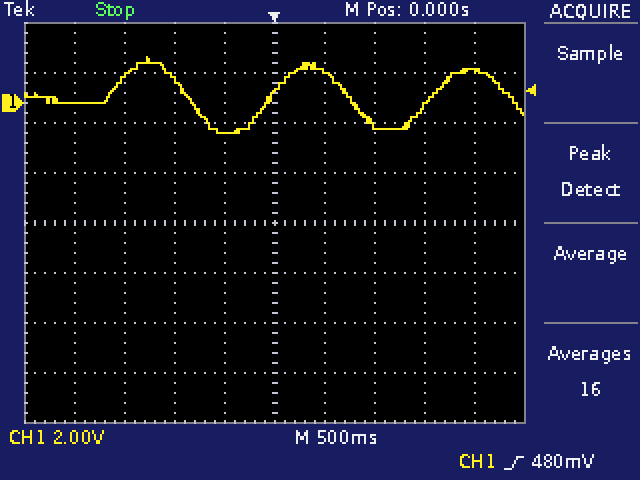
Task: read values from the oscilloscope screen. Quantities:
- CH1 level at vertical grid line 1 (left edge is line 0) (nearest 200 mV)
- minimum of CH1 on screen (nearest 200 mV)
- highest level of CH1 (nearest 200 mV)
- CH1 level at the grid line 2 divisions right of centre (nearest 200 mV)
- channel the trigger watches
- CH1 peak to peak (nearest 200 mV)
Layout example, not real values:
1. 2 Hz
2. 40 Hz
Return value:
1. 0.0 V
2. -1.2 V
3. 1.8 V
4. -800 mV
5. CH1
6. 3.0 V
